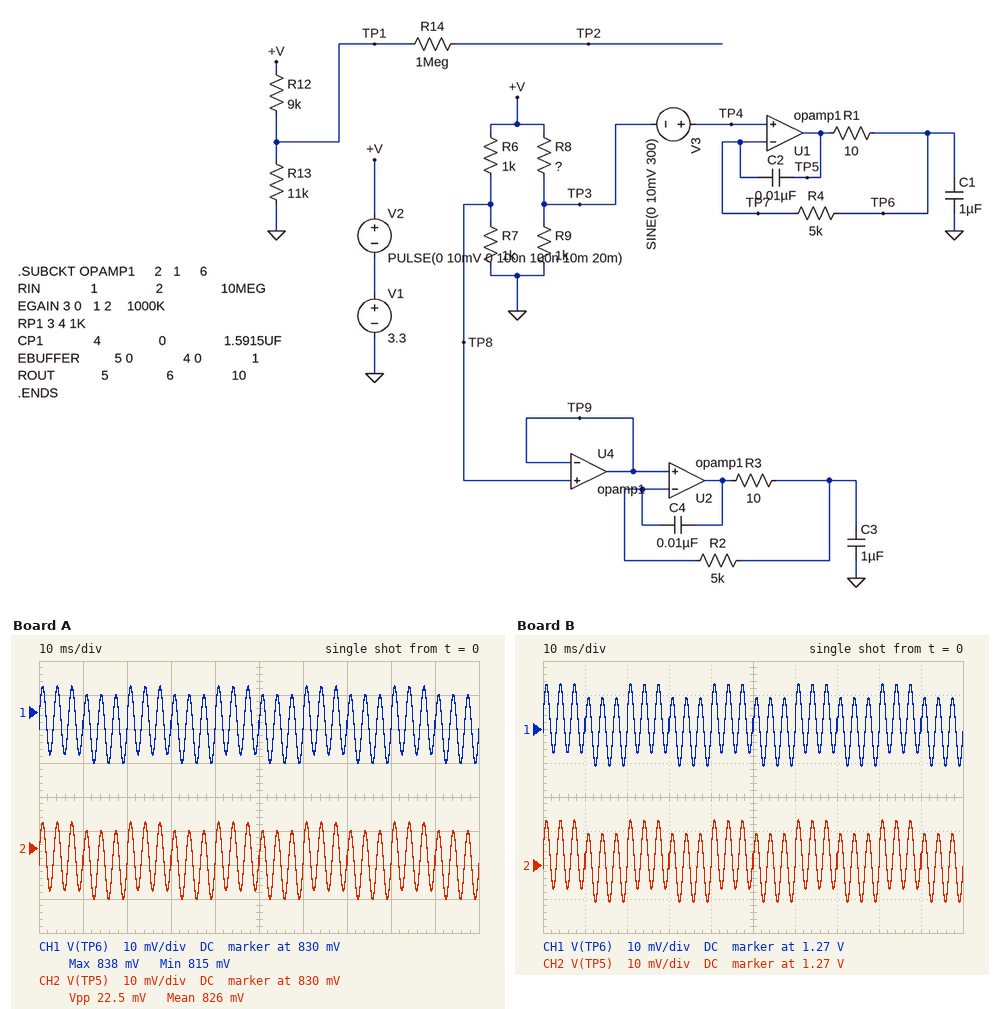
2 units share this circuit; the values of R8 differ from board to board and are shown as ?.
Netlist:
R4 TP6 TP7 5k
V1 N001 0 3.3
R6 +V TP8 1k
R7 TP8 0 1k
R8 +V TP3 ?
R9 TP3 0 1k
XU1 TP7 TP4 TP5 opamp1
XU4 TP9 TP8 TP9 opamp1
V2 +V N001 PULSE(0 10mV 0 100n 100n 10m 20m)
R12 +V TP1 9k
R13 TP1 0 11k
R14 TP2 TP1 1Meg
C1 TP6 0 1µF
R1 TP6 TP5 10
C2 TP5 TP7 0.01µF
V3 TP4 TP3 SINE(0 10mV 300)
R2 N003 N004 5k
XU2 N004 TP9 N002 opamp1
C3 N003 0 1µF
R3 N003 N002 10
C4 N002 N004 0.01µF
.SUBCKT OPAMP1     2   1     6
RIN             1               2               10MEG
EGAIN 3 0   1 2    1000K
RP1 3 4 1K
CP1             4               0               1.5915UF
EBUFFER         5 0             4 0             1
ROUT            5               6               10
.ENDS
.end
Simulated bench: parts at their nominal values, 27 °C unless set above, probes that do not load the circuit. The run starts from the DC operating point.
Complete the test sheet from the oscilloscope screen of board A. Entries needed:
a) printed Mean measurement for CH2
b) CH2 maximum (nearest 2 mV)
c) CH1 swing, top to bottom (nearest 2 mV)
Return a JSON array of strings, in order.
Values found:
["826 mV", "838 mV", "22 mV"]
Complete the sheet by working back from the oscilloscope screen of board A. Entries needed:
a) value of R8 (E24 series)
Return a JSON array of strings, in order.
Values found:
["3 kΩ"]
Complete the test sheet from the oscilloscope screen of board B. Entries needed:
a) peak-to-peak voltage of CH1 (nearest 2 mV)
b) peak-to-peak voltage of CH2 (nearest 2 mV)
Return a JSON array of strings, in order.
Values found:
["24 mV", "24 mV"]
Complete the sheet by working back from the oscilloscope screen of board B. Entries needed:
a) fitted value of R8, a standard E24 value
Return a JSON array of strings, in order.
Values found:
["1.6 kΩ"]
